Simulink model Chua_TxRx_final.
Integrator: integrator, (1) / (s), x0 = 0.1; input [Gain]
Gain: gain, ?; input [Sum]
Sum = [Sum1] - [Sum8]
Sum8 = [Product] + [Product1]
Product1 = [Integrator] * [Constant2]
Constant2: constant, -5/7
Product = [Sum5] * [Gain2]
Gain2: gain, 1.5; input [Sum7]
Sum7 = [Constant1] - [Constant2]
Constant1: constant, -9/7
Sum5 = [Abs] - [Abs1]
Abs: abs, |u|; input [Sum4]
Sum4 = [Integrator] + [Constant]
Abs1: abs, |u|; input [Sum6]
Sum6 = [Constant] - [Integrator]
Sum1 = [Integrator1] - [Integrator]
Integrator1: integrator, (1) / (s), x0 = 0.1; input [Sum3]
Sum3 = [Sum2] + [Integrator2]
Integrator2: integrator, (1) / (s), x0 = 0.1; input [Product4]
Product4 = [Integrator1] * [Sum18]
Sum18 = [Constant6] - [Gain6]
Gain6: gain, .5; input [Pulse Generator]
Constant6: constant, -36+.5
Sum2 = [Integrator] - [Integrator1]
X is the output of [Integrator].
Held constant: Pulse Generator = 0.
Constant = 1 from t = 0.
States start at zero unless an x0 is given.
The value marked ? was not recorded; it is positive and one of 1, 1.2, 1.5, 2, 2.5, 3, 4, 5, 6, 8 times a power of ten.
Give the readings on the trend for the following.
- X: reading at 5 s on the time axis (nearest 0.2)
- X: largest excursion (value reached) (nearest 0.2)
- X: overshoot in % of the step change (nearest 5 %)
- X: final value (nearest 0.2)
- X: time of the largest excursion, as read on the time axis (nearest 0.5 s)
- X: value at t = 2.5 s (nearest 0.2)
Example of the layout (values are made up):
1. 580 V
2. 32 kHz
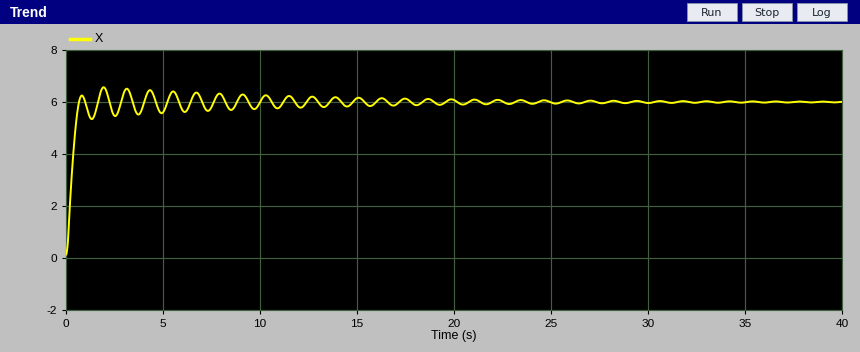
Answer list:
1. 5.6
2. 6.6
3. 10 %
4. 6.0
5. 2.0 s
6. 5.4
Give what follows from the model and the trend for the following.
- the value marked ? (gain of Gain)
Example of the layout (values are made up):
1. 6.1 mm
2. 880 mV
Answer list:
1. 10
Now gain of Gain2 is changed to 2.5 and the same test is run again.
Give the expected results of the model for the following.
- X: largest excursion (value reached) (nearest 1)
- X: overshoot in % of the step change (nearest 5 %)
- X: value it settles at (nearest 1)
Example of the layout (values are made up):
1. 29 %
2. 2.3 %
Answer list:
1. 11
2. 10 %
3. 10
